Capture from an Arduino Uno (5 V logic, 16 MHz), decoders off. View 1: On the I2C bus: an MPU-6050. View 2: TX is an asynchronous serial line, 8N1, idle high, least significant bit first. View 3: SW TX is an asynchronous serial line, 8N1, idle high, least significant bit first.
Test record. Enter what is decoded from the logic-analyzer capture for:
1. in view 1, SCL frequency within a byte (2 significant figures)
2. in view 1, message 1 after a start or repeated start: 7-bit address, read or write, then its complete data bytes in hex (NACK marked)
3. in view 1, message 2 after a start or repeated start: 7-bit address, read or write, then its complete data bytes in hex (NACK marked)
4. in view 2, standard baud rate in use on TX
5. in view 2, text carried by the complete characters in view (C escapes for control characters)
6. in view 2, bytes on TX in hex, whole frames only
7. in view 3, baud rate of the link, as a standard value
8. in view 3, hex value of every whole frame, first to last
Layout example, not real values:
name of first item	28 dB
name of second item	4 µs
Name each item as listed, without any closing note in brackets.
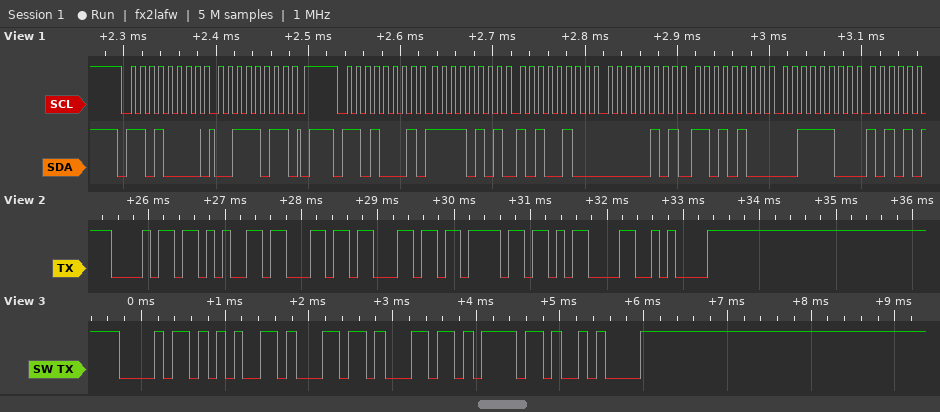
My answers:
in view 1, SCL frequency within a byte	100 kHz
in view 1, message 1 after a start or repeated start: 7-bit address, read or write, then its complete data bytes in hex	0x68 write: 3B
in view 1, message 2 after a start or repeated start: 7-bit address, read or write, then its complete data bytes in hex	0x68 read: F5 A4 05 D4 3C
in view 2, standard baud rate in use on TX	9600 baud
in view 2, text carried by the complete characters in view	"hello\r\n"
in view 2, bytes on TX in hex, whole frames only	68 65 6C 6C 6F 0D 0A
in view 3, baud rate of the link, as a standard value	9600 baud
in view 3, hex value of every whole frame, first to last	68 65 6C 6C 6F 0A
